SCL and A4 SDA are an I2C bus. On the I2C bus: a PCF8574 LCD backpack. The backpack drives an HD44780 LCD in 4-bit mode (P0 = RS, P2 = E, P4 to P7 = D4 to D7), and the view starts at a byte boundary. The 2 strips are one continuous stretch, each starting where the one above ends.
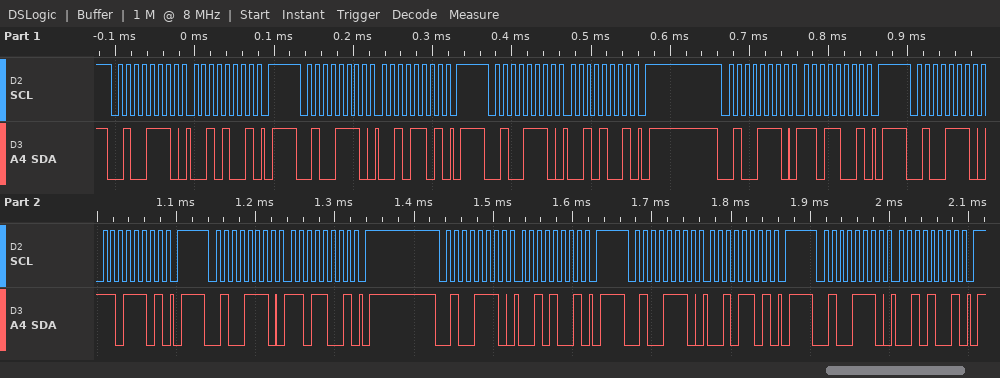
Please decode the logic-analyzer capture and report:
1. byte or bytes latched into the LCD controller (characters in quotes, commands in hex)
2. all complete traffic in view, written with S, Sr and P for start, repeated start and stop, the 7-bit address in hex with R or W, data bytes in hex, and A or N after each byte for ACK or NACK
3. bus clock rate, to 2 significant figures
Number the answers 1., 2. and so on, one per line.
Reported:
1. '-'
2. S 27W A 29 A P S 27W A 2D A P S 27W A 29 A P S 27W A D9 A P S 27W A DD A P S 27W A D9 A P S 27W A 29 A P S 27W A 2D A P S 27W A 29 A P
3. 100 kHz
